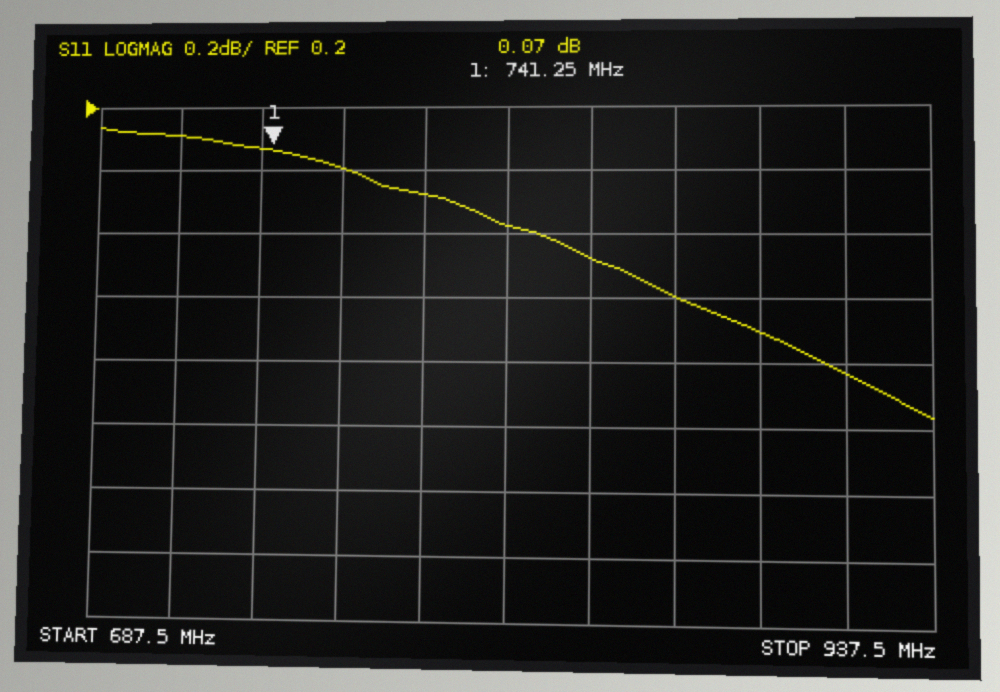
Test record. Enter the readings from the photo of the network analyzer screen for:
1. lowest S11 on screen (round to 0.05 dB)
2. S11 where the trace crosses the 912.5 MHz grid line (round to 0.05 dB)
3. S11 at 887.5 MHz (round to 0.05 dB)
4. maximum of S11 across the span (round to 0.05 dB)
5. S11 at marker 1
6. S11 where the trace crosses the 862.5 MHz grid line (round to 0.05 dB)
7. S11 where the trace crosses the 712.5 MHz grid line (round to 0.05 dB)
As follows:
-0.75 dB
-0.65 dB
-0.50 dB
0.15 dB
0.07 dB
-0.40 dB
0.10 dB
